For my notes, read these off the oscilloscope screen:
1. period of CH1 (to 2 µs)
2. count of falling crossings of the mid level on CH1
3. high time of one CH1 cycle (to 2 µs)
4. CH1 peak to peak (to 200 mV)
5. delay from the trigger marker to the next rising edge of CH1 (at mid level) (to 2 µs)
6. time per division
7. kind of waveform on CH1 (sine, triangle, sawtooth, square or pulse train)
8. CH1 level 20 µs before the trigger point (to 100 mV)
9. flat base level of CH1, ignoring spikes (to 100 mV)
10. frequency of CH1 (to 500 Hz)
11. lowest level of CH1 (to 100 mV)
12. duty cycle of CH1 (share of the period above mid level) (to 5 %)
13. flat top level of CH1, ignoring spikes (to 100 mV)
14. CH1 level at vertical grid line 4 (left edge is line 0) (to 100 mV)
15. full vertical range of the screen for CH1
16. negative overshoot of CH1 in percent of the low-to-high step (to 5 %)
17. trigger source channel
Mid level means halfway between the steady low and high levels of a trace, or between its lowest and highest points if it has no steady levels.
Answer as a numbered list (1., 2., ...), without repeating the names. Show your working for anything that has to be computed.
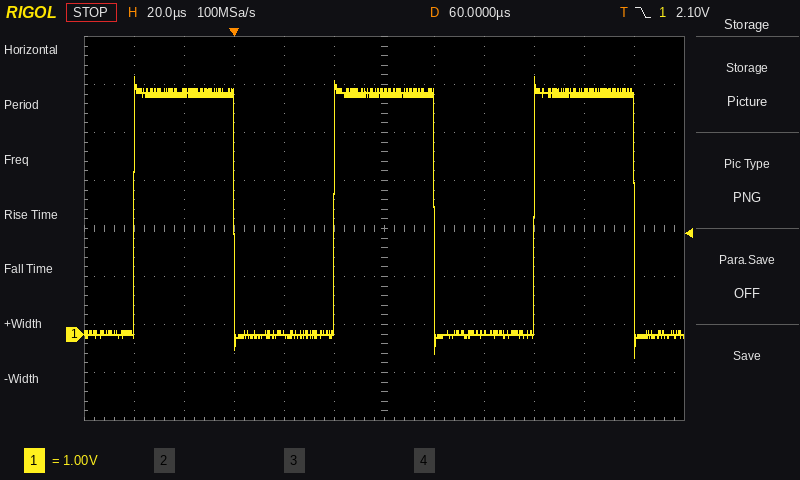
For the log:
1. 80 µs
2. 3
3. 40 µs
4. 5.8 V
5. 40 µs
6. 20 µs
7. square
8. 5.0 V
9. 0.0 V
10. 1 / 80 µs ≈ 12.5 kHz
11. -500 mV
12. 40 µs / 80 µs ≈ 50 %
13. 5.0 V
14. 0.0 V
15. 8 V
16. 10 %
17. CH1
